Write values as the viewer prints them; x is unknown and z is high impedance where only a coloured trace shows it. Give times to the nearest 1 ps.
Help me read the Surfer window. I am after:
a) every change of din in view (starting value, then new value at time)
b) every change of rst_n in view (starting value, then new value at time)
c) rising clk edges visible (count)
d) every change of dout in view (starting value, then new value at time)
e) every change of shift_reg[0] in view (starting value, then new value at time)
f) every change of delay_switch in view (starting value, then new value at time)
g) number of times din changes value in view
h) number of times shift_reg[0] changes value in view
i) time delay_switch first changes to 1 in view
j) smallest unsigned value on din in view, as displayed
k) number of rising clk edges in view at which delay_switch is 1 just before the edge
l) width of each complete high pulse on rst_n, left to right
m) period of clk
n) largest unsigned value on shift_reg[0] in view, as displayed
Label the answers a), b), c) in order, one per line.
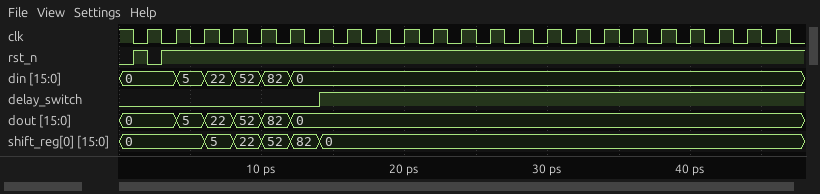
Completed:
a) 0, 5 at 4 ps, 22 at 6 ps, 52 at 8 ps, 82 at 10 ps, 0 at 12 ps
b) 0, 1 at 1 ps, 0 at 2 ps, 1 at 3 ps
c) 23
d) 0, 5 at 4 ps, 22 at 6 ps, 52 at 8 ps, 82 at 10 ps, 0 at 12 ps
e) 0, 5 at 6 ps, 22 at 8 ps, 52 at 10 ps, 82 at 12 ps, 0 at 14 ps
f) 0, 1 at 14 ps
g) 5
h) 5
i) 14 ps
j) 0
k) 16
l) 1 ps
m) 2 ps
n) 82
